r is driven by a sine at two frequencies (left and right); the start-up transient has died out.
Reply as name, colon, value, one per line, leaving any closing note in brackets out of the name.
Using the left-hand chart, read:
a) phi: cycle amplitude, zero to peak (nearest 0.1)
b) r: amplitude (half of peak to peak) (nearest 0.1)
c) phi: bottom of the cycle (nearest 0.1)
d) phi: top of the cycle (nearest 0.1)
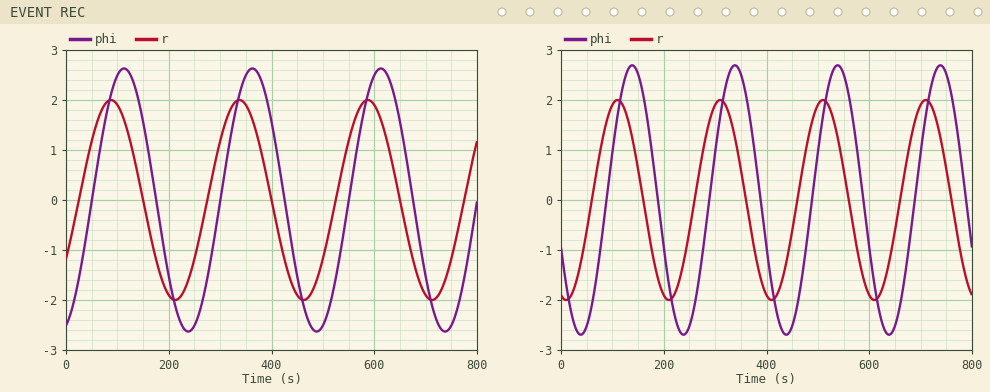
phi: cycle amplitude, zero to peak: 2.6
r: amplitude (half of peak to peak): 2.0
phi: bottom of the cycle: -2.6
phi: top of the cycle: 2.6
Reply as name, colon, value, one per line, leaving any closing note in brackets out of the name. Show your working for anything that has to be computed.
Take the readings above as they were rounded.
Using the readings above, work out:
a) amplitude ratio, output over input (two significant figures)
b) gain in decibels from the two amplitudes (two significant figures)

amplitude ratio, output over input: 2.6 / 2 = 1.3
gain in decibels from the two amplitudes: 20 log10(2.6 / 2) = 2.3 dB
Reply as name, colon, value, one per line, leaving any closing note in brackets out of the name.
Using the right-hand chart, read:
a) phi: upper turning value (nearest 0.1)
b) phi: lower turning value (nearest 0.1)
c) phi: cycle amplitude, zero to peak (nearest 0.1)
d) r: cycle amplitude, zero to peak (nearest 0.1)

phi: upper turning value: 2.7
phi: lower turning value: -2.7
phi: cycle amplitude, zero to peak: 2.7
r: cycle amplitude, zero to peak: 2.0
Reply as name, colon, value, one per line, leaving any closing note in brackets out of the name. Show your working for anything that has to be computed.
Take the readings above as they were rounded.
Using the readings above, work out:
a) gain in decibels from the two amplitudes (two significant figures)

gain in decibels from the two amplitudes: 20 log10(2.7 / 2) = 2.6 dB
